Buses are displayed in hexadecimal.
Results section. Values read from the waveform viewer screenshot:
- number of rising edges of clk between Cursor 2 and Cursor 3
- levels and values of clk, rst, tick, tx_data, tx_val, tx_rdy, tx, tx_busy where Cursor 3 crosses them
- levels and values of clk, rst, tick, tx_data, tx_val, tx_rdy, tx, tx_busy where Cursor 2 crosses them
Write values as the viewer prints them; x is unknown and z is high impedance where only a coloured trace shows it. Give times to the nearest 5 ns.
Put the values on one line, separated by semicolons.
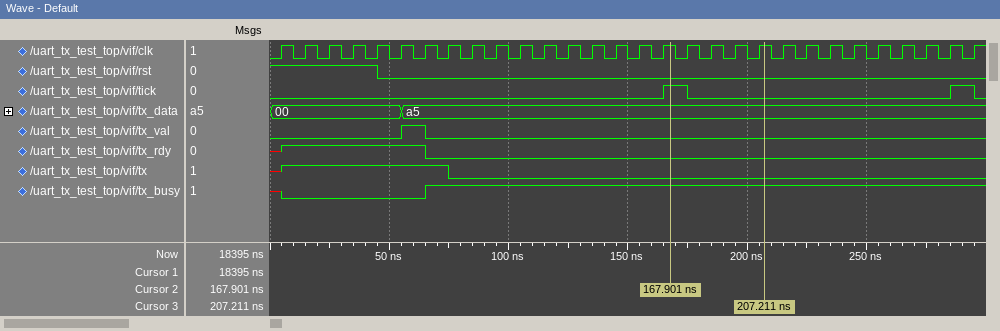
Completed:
4; clk=1, rst=0, tick=0, tx_data=a5, tx_val=0, tx_rdy=0, tx=0, tx_busy=1; clk=1, rst=0, tick=1, tx_data=a5, tx_val=0, tx_rdy=0, tx=0, tx_busy=1
